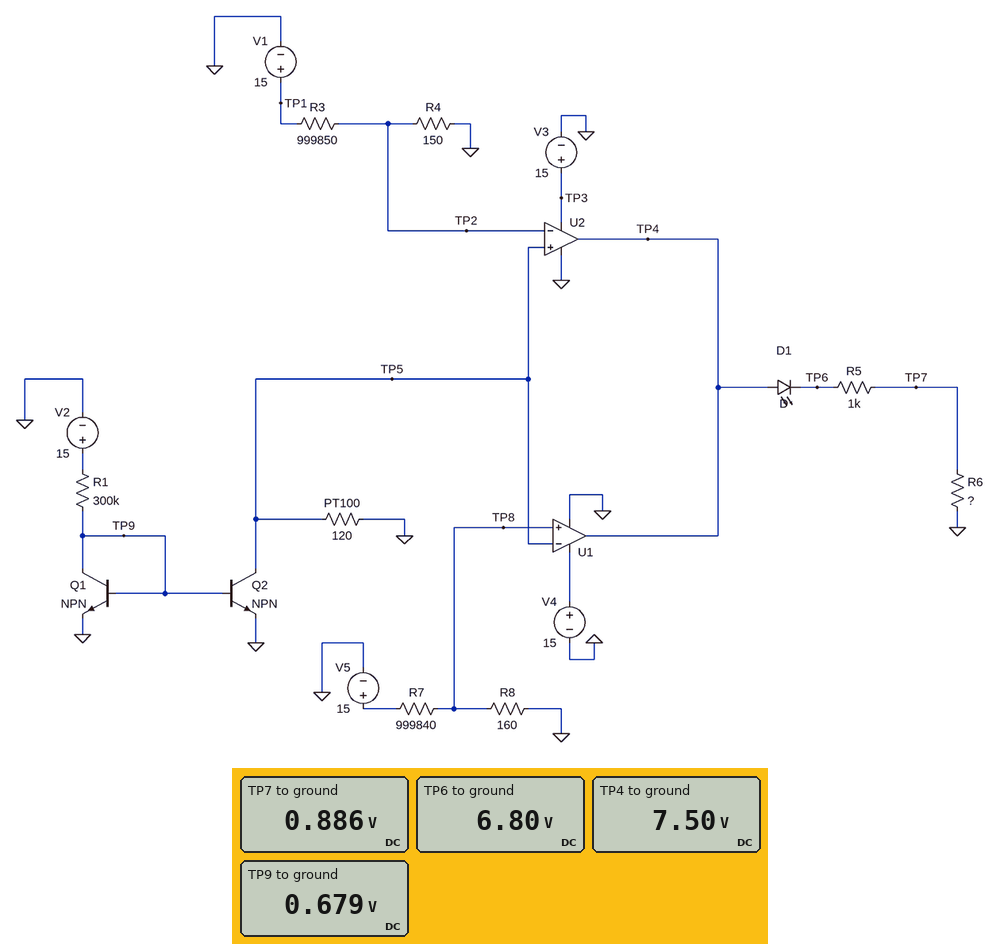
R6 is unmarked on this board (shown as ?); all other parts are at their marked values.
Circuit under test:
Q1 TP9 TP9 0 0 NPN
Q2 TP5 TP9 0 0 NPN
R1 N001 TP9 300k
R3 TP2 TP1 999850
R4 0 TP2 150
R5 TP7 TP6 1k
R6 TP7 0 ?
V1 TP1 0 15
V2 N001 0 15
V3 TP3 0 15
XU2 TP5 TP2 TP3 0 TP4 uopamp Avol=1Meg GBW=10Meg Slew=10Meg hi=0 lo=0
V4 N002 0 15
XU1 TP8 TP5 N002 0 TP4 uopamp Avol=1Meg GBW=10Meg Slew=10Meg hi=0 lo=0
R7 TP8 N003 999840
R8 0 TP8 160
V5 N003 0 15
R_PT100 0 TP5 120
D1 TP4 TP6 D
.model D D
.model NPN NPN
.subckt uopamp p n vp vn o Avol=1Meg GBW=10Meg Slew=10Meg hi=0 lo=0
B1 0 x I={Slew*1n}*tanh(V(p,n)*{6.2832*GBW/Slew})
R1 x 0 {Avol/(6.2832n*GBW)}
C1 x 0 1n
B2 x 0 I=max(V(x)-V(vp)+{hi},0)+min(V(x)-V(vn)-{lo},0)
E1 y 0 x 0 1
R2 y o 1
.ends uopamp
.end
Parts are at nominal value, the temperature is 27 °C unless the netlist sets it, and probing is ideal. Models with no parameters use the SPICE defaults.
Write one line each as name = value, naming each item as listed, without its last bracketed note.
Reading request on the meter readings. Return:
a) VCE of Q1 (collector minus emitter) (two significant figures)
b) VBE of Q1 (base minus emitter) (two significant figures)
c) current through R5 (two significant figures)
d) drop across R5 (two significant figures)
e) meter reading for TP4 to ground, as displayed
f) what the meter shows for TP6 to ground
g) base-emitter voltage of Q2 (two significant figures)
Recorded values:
VCE of Q1 (collector minus emitter) = 680 mV
VBE of Q1 (base minus emitter) = 680 mV
current through R5 = 5.9 mA
drop across R5 = 5.9 V
meter reading for TP4 to ground, as displayed = 7.50 V
what the meter shows for TP6 to ground = 6.80 V
base-emitter voltage of Q2 = 680 mV
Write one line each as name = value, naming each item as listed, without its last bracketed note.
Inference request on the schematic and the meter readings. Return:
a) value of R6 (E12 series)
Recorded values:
value of R6 = 150 Ω
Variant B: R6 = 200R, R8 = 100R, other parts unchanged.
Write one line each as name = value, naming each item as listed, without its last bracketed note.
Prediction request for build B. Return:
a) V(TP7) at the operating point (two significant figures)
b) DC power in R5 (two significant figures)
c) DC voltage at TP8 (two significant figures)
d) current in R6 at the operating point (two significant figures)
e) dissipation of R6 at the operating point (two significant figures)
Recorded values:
V(TP7) at the operating point = 1.1 V
DC power in R5 = 32 mW
DC voltage at TP8 = 1.5 mV
current in R6 at the operating point = 5.7 mA
dissipation of R6 at the operating point = 6.4 mW
